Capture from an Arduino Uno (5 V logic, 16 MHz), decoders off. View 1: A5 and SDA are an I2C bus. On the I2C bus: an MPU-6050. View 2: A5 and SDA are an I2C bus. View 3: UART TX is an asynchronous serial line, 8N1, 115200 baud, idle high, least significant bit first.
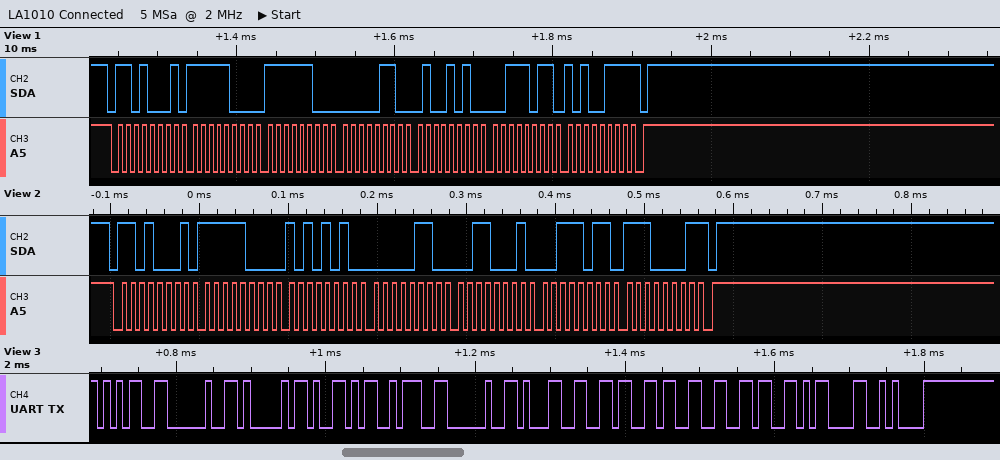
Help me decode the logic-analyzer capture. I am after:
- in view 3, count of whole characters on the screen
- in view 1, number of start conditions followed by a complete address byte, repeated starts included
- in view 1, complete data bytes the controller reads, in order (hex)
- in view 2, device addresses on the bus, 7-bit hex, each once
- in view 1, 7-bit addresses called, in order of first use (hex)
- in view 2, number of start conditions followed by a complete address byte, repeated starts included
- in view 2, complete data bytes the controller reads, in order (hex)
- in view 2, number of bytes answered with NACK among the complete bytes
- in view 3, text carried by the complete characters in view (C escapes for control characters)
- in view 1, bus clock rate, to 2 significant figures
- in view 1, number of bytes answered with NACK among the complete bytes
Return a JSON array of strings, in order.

["12", "1", "F8 FC 06 4A 3B A7", "0x68", "0x68", "1", "F8 AA 06 31 3B E1", "1", "\"5 AY: 1636\\r\\n\"", "100 kHz", "1"]
